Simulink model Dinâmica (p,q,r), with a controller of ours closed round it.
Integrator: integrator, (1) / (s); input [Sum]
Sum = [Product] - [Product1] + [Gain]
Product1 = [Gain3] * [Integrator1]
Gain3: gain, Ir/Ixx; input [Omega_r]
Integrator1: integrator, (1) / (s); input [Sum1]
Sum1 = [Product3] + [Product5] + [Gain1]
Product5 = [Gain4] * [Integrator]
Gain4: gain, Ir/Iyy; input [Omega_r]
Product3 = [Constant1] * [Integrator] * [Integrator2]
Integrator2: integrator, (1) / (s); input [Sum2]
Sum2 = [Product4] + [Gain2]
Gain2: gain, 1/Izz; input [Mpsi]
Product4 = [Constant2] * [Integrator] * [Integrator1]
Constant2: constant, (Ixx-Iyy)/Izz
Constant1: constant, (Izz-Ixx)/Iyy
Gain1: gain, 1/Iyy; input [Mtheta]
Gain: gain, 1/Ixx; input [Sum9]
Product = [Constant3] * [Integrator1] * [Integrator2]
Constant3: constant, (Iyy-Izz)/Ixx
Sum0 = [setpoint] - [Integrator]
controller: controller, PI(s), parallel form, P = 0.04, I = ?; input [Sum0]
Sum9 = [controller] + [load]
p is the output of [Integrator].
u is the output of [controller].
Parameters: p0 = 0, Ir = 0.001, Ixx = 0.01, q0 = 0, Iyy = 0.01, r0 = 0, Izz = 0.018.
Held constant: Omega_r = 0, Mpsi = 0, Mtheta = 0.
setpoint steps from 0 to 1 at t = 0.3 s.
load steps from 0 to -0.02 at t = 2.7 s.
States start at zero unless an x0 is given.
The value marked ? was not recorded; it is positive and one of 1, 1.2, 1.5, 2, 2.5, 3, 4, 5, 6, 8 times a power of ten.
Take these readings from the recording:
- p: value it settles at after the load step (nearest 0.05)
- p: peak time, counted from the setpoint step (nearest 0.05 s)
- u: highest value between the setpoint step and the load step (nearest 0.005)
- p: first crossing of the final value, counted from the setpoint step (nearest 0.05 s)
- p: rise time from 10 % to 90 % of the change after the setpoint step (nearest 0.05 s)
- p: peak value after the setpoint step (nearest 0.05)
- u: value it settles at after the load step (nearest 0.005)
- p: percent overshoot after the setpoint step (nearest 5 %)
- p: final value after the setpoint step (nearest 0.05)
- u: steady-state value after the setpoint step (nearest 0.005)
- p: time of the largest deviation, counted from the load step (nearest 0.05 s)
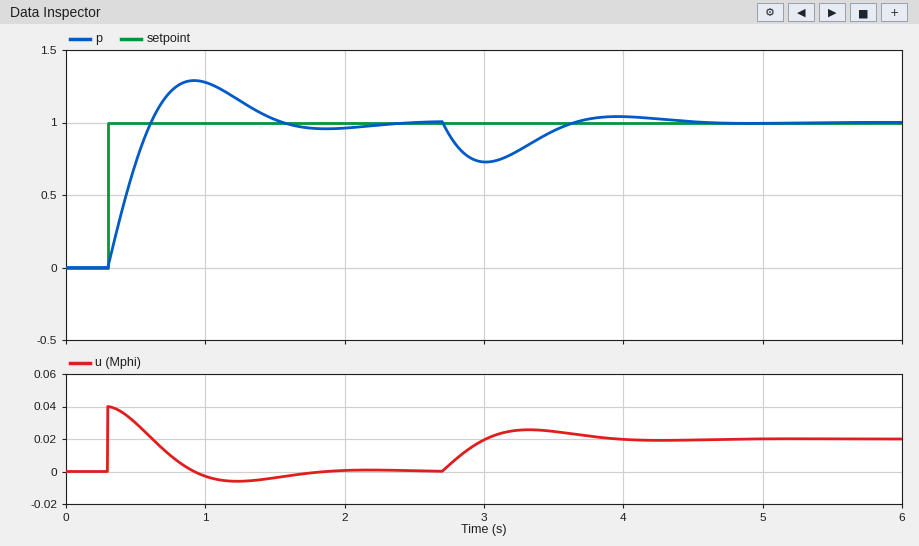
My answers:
1.00
0.60 s
0.040
0.30 s
0.25 s
1.30
0.020
30 %
1.00
0.000
0.30 s
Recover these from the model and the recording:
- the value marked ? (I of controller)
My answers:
0.15
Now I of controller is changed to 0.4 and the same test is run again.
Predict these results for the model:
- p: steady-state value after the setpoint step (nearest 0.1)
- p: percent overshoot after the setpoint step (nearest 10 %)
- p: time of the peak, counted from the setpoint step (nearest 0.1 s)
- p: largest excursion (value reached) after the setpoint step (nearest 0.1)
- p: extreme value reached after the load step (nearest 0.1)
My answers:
1.0
40 %
0.4 s
1.4
0.8
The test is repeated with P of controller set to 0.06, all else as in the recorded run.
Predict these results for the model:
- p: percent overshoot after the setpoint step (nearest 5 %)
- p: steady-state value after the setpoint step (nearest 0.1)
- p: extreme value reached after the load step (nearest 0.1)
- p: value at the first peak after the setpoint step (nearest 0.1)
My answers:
20 %
1.0
0.8
1.2
